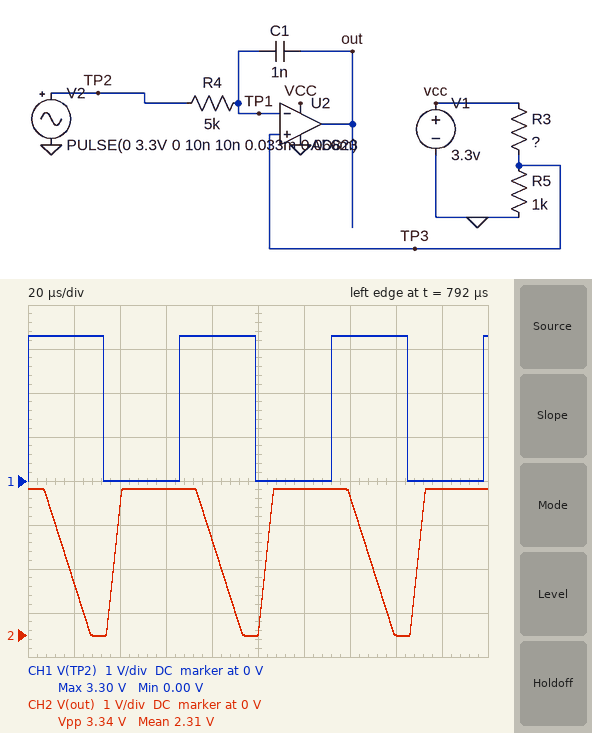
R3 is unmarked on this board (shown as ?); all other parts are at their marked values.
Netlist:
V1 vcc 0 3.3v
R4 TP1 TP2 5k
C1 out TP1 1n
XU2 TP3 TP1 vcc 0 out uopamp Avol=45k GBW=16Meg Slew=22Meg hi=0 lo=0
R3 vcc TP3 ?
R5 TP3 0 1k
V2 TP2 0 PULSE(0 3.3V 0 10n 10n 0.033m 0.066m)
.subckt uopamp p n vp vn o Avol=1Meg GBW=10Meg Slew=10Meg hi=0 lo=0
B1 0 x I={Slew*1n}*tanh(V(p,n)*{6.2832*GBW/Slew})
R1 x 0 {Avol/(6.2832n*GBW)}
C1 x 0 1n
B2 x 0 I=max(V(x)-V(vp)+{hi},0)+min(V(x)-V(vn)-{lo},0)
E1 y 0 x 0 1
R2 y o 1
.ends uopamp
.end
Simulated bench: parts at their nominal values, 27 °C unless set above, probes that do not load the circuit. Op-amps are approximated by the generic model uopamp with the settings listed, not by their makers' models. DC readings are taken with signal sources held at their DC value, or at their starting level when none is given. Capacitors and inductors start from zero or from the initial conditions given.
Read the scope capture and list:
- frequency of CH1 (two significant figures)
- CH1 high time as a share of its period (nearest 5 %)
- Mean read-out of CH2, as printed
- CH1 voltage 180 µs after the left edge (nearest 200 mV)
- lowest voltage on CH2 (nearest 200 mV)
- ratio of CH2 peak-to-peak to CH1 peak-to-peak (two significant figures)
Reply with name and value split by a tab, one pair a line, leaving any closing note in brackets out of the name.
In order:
frequency of CH1	15 kHz
CH1 high time as a share of its period	50 %
Mean read-out of CH2, as printed	2.31 V
CH1 voltage 180 µs after the left edge	0 V
lowest voltage on CH2	0 V
ratio of CH2 peak-to-peak to CH1 peak-to-peak	1.0
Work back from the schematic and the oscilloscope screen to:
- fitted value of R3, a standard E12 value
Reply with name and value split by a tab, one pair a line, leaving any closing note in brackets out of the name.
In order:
fitted value of R3, a standard E12 value	330 Ω
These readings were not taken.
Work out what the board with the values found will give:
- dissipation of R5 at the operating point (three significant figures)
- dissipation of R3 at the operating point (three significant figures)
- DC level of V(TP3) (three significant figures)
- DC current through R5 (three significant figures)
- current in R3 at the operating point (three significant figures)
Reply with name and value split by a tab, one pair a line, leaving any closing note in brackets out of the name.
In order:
dissipation of R5 at the operating point	6.16 mW
dissipation of R3 at the operating point	2.03 mW
DC level of V(TP3)	2.48 V
DC current through R5	2.48 mA
current in R3 at the operating point	2.48 mA
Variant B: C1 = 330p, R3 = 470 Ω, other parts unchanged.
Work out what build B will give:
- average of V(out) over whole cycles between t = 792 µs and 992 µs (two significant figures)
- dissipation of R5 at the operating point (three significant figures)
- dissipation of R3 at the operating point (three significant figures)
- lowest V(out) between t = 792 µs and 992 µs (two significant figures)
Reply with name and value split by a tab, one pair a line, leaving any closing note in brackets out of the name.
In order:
average of V(out) over whole cycles between t = 792 µs and 992 µs	1.8 V
dissipation of R5 at the operating point	5.04 mW
dissipation of R3 at the operating point	2.37 mW
lowest V(out) between t = 792 µs and 992 µs	-23 mV
